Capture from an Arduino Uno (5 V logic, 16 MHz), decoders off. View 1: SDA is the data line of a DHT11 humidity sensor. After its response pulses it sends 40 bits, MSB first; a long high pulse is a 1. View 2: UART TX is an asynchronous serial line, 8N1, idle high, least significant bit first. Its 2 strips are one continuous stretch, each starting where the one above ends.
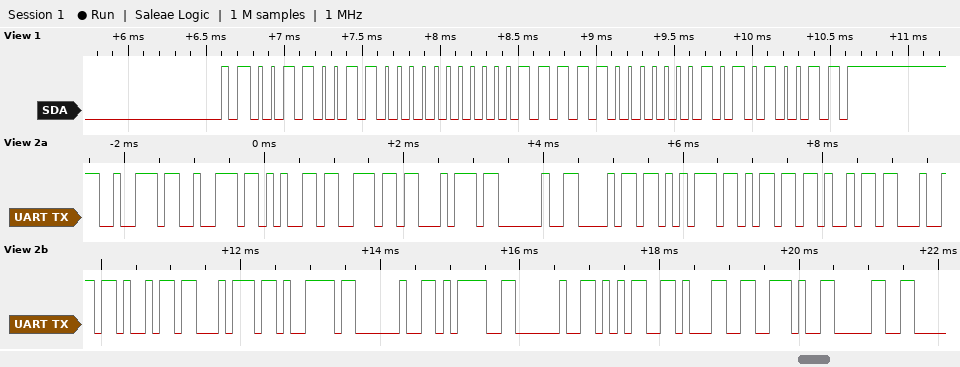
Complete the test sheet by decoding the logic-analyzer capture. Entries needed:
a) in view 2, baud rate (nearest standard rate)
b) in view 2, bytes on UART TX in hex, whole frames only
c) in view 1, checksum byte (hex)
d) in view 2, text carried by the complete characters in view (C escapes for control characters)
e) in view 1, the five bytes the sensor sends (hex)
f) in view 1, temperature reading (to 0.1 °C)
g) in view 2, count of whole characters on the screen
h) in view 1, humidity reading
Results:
9600 baud
72 72 65 6E 74 20 68 75 6D 69 64 69 74 79 20 3D 20 35 31 2E 30
0x53
"rrent humidity = 51.0"
33 00 1F 01 53
31.1 °C
21
51 %
